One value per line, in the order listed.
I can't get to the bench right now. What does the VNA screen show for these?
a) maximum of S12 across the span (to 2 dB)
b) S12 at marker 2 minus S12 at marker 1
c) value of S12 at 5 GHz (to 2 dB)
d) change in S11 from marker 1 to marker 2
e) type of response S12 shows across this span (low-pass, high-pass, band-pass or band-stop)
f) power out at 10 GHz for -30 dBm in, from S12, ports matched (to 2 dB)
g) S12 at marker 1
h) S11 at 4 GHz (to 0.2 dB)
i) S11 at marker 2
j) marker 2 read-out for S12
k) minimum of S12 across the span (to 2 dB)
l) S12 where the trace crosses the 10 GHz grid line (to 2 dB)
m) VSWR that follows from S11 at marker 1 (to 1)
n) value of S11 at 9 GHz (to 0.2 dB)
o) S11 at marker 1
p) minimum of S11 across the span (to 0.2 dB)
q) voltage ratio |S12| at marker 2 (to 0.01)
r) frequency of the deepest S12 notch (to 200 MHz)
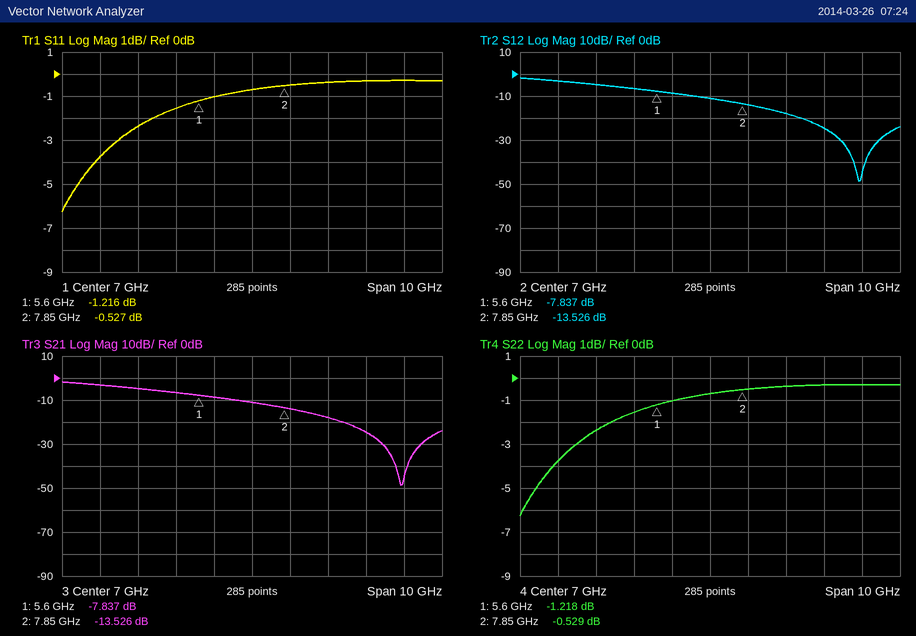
-2 dB
-5.689 dB
-6 dB
0.689 dB
low-pass
-54 dBm
-7.837 dB
-2.4 dB
-0.527 dB
-13.526 dB
-48 dB
-24 dB
14
-0.4 dB
-1.216 dB
-6.2 dB
0.21
11.0 GHz
